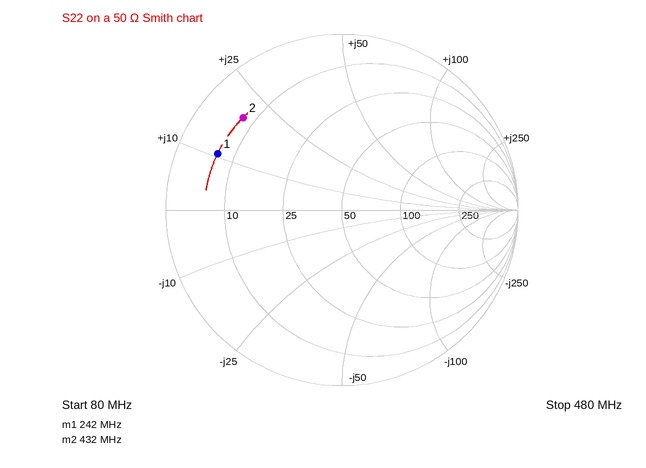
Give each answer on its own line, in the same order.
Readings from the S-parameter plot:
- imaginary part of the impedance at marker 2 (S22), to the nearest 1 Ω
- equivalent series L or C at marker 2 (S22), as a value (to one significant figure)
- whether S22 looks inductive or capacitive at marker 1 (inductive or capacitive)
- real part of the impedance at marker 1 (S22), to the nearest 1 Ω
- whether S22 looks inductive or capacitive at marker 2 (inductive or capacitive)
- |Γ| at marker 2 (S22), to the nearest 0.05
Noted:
+19 Ω
7 nH
inductive
7 Ω
inductive
0.75
